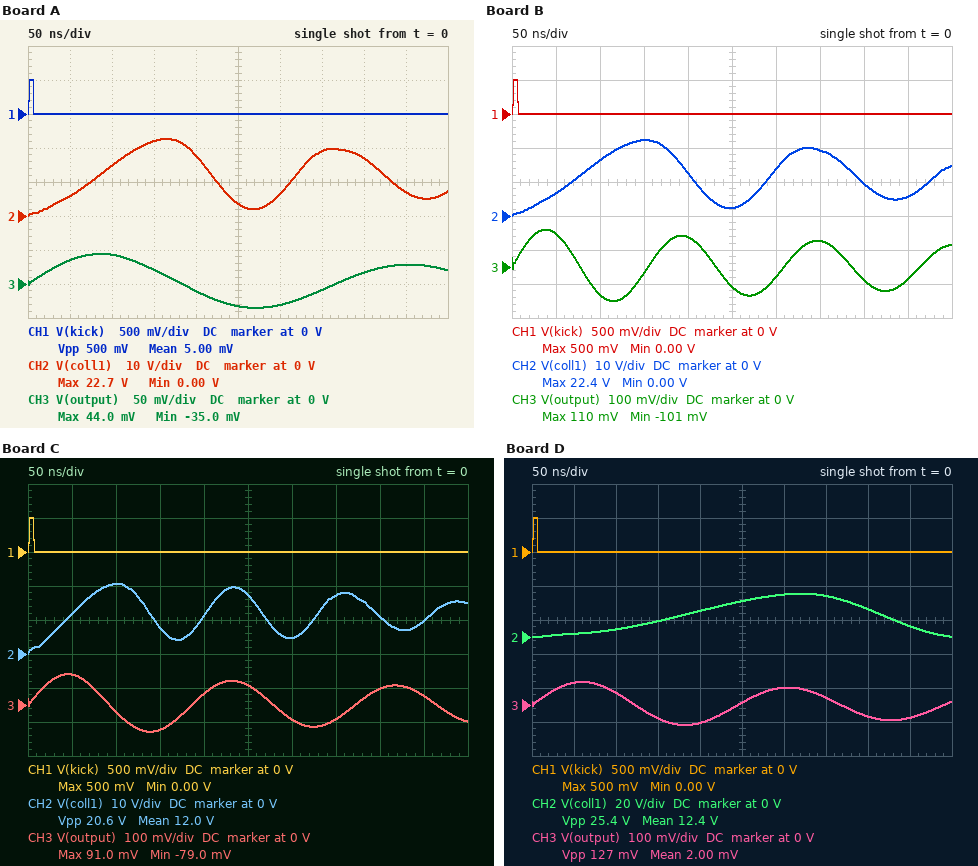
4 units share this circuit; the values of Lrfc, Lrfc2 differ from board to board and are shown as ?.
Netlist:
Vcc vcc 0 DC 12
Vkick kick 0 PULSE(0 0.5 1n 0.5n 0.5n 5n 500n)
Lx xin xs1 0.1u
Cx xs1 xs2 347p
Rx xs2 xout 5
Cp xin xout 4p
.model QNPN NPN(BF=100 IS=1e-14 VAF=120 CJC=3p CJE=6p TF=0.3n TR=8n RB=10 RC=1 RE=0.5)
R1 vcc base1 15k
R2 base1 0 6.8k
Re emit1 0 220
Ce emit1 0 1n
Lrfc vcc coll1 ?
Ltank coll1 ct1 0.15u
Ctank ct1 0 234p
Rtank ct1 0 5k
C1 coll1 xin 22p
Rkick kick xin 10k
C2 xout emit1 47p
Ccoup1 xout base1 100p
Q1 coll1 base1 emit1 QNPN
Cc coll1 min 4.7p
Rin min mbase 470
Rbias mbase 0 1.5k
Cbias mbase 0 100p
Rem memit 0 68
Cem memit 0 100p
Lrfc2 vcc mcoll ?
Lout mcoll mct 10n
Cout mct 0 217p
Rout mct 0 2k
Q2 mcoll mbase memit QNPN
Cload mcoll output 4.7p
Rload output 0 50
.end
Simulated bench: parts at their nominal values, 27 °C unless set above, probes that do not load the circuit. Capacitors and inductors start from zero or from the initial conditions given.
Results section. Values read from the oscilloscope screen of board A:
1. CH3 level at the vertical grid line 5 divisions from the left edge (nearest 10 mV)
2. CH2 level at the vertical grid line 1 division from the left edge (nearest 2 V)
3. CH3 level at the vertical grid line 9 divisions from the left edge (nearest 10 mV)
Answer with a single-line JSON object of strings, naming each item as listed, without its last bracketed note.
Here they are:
{"CH3 level at the vertical grid line 5 divisions from the left edge": "-30 mV", "CH2 level at the vertical grid line 1 division from the left edge": "6 V", "CH3 level at the vertical grid line 9 divisions from the left edge": "30 mV"}
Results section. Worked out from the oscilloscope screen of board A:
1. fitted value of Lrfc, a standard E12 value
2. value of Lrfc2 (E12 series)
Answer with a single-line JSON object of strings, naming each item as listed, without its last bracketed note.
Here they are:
{"fitted value of Lrfc, a standard E12 value": "3.9 µH", "value of Lrfc2": "15 µH"}
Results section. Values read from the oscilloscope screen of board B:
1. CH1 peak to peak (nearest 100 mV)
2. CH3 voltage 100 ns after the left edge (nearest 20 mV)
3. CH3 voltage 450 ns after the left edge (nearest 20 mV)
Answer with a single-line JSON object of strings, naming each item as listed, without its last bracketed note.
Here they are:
{"CH1 peak to peak": "500 mV", "CH3 voltage 100 ns after the left edge": "-80 mV", "CH3 voltage 450 ns after the left edge": "-40 mV"}
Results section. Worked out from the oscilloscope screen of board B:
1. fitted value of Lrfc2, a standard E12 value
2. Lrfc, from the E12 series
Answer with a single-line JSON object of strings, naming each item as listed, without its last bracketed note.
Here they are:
{"fitted value of Lrfc2, a standard E12 value": "2.7 µH", "Lrfc, from the E12 series": "3.3 µH"}
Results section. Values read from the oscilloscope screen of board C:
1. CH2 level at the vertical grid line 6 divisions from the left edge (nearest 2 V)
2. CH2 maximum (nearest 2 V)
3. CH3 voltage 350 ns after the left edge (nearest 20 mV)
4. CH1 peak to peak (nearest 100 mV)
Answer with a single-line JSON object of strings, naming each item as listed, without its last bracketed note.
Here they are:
{"CH2 level at the vertical grid line 6 divisions from the left edge": "4 V", "CH2 maximum": "20 V", "CH3 voltage 350 ns after the left edge": "-40 mV", "CH1 peak to peak": "500 mV"}
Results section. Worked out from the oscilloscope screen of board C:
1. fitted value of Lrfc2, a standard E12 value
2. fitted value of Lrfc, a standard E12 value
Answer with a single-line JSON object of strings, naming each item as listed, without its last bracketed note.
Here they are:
{"fitted value of Lrfc2, a standard E12 value": "3.9 µH", "fitted value of Lrfc, a standard E12 value": "1.5 µH"}
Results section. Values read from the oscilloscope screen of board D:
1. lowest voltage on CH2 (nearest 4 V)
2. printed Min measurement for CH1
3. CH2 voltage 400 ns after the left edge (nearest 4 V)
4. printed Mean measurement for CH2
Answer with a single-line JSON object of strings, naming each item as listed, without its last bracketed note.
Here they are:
{"lowest voltage on CH2": "0 V", "printed Min measurement for CH1": "0.00 V", "CH2 voltage 400 ns after the left edge": "16 V", "printed Mean measurement for CH2": "12.4 V"}
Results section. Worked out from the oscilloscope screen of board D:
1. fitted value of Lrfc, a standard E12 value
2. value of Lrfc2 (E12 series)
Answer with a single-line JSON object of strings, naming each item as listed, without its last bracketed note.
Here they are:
{"fitted value of Lrfc, a standard E12 value": "15 µH", "value of Lrfc2": "6.8 µH"}
